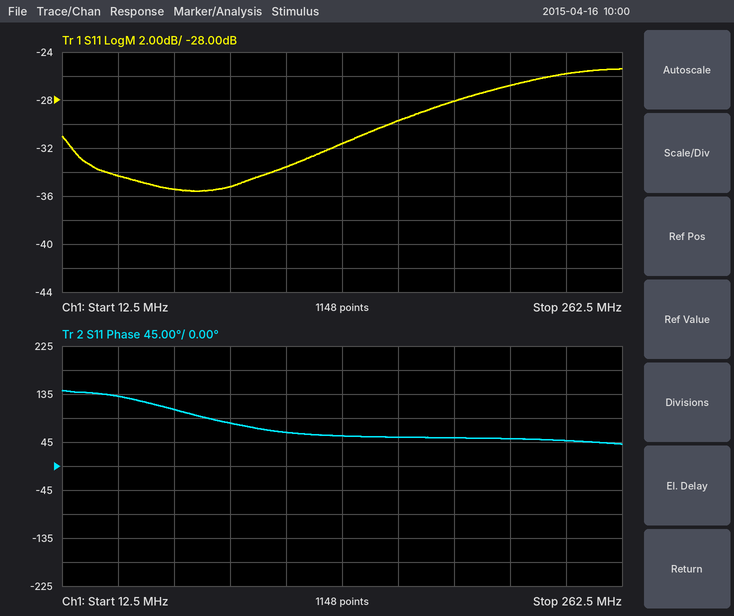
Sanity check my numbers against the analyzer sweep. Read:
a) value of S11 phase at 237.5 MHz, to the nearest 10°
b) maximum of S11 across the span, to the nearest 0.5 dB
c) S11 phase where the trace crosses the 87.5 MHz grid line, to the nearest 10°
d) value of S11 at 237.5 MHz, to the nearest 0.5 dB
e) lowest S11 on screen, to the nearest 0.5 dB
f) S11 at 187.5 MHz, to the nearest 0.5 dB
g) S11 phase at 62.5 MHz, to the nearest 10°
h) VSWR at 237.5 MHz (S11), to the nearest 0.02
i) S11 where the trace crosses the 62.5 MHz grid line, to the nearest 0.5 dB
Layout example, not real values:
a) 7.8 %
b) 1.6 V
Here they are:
a) 50°
b) -25.5 dB
c) 80°
d) -26.0 dB
e) -35.5 dB
f) -28.0 dB
g) 110°
h) 1.10
i) -35.5 dB
